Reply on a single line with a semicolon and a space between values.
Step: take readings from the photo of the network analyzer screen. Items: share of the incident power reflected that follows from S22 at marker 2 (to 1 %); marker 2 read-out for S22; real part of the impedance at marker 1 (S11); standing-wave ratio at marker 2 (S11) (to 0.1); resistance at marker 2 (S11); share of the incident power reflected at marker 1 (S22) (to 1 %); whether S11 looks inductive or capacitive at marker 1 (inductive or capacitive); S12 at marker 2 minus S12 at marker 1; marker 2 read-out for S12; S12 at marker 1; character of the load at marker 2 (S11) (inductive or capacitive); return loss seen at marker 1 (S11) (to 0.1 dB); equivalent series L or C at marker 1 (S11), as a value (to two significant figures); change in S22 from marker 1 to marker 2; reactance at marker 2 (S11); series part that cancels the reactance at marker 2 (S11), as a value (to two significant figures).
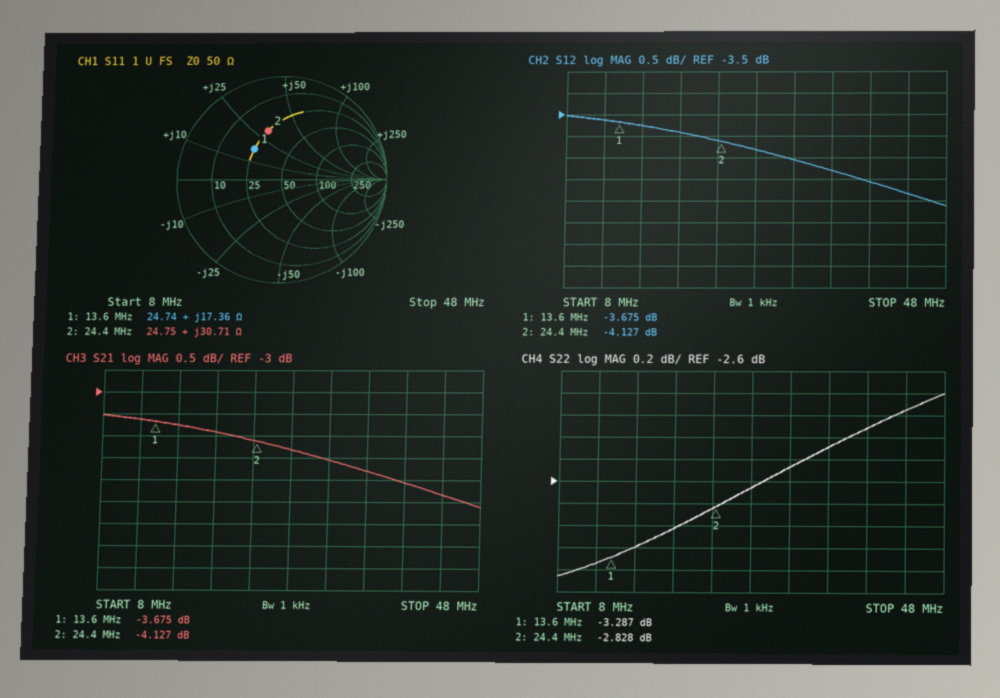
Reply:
52 %; -2.828 dB; 24.74 Ω; 2.9; 24.75 Ω; 47 %; inductive; -0.452 dB; -4.127 dB; -3.675 dB; inductive; 8.0 dB; 200 nH; 0.459 dB; +30.71 Ω; 210 pF
